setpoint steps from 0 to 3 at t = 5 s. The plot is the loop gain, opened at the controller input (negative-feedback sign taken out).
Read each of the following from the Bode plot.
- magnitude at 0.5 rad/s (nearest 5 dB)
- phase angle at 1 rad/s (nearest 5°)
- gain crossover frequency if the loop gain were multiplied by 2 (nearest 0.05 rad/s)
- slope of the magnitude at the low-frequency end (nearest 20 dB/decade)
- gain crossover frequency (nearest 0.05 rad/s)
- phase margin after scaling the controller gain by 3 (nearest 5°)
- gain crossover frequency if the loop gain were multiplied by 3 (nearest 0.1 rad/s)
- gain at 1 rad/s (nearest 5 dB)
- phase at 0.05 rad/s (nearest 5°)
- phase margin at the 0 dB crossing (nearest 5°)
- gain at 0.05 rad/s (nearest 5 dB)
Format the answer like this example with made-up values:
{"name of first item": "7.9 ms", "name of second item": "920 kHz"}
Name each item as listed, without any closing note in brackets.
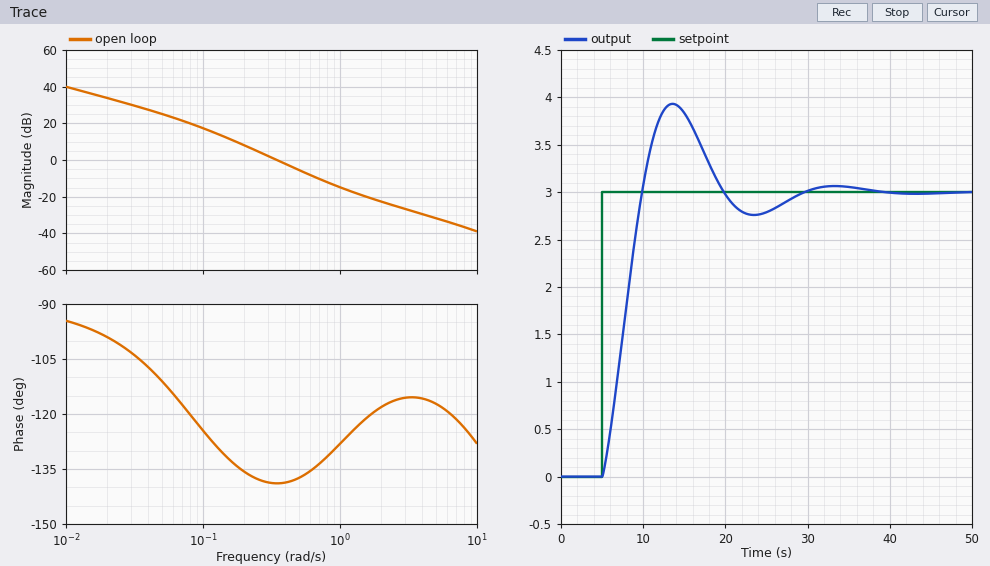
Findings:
{"magnitude at 0.5 rad/s": "-5 dB", "phase angle at 1 rad/s": "-130°", "gain crossover frequency if the loop gain were multiplied by 2": "0.50 rad/s", "slope of the magnitude at the low-frequency end": "-20 dB/decade", "gain crossover frequency": "0.35 rad/s", "phase margin after scaling the controller gain by 3": "45°", "gain crossover frequency if the loop gain were multiplied by 3": "0.7 rad/s", "gain at 1 rad/s": "-15 dB", "phase at 0.05 rad/s": "-110°", "phase margin at the 0 dB crossing": "40°", "gain at 0.05 rad/s": "25 dB"}
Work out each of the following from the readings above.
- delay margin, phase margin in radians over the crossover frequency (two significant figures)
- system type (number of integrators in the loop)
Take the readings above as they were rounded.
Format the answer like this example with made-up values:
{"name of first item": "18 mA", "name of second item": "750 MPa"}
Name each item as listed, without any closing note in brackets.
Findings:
{"delay margin, phase margin in radians over the crossover frequency": "2.0 s", "system type": "1"}
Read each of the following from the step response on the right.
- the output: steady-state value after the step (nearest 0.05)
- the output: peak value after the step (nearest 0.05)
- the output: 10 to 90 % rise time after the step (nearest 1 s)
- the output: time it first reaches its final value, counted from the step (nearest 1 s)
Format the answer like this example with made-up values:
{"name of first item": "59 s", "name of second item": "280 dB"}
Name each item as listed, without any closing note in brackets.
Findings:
{"the output: steady-state value after the step": "3.00", "the output: peak value after the step": "3.95", "the output: 10 to 90 % rise time after the step": "4 s", "the output: time it first reaches its final value, counted from the step": "5 s"}
